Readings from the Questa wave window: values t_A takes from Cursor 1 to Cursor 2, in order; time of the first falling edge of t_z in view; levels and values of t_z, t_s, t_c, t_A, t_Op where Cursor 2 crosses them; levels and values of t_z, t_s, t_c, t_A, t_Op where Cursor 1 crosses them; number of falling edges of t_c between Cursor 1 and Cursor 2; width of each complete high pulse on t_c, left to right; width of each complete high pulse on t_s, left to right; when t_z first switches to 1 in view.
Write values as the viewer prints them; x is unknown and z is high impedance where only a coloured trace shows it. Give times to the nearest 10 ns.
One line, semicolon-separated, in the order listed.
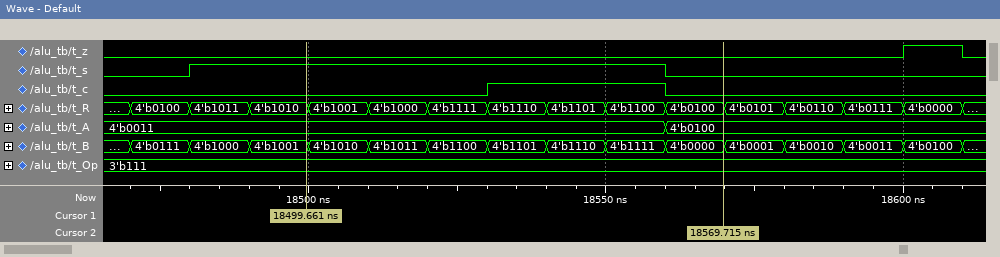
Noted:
4'b0011, 4'b0100; 18610 ns; t_z=0, t_s=0, t_c=0, t_A=4'b0100, t_Op=3'b111; t_z=0, t_s=1, t_c=0, t_A=4'b0011, t_Op=3'b111; 1; 30 ns; 80 ns; 18600 ns
